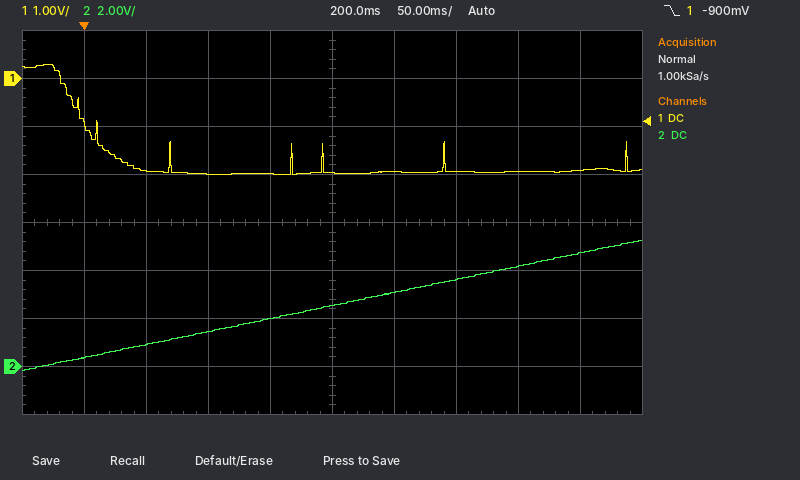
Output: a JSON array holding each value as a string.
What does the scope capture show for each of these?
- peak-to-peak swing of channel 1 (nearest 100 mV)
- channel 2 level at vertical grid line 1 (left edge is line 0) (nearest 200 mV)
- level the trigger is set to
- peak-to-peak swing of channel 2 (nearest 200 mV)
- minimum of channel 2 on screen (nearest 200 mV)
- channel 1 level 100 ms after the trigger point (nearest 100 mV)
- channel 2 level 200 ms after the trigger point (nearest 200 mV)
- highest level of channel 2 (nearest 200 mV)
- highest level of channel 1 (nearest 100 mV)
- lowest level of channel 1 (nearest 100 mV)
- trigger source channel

["2.3 V", "400 mV", "-900 mV", "5.4 V", "-200 mV", "-2.0 V", "2.6 V", "5.2 V", "300 mV", "-2.0 V", "channel 1"]
